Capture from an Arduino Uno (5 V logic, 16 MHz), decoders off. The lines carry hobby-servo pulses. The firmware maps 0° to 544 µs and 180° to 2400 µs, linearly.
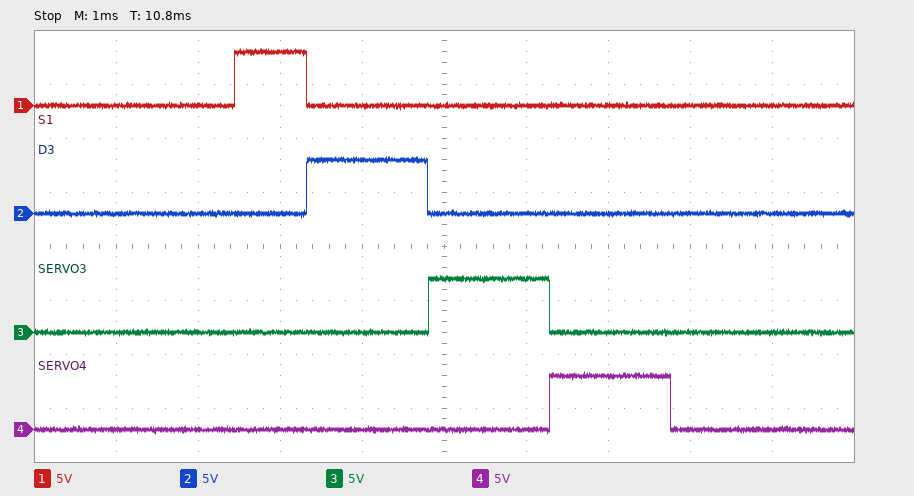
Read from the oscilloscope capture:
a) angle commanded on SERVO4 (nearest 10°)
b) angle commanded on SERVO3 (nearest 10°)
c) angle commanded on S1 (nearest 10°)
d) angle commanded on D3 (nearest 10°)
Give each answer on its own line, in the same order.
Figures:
90°
90°
30°
90°
